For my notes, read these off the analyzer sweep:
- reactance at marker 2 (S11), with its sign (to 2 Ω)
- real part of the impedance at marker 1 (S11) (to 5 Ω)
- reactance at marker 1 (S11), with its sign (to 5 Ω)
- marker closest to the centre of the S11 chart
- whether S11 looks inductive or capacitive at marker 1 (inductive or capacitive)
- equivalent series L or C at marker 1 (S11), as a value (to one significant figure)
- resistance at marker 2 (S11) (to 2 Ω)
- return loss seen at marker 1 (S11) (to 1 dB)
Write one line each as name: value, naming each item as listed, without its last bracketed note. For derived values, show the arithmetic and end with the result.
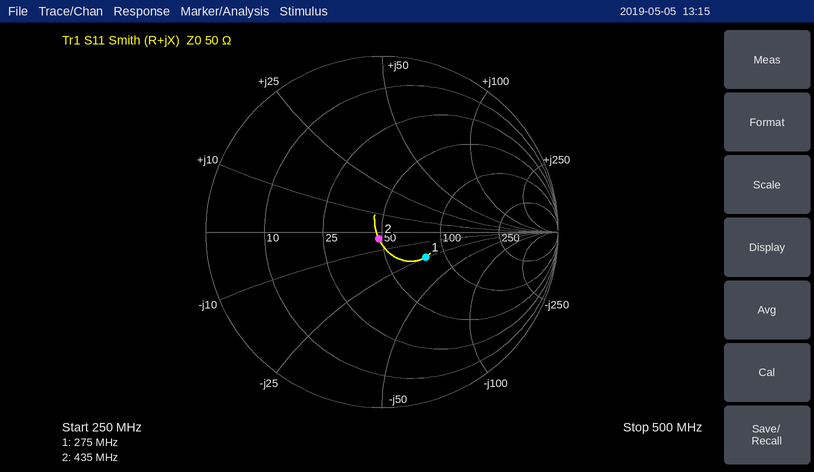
reactance at marker 2 (S11), with its sign: -4 Ω
real part of the impedance at marker 1 (S11): 80 Ω
reactance at marker 1 (S11), with its sign: -25 Ω
marker closest to the centre of the S11 chart: marker 2
whether S11 looks inductive or capacitive at marker 1: capacitive
equivalent series L or C at marker 1 (S11), as a value: C = 1/(2π × 275 MHz × 25 Ω) ≈ 23.1 pF, so 20 pF to one significant figure
resistance at marker 2 (S11): 48 Ω
return loss seen at marker 1 (S11): 11 dB
